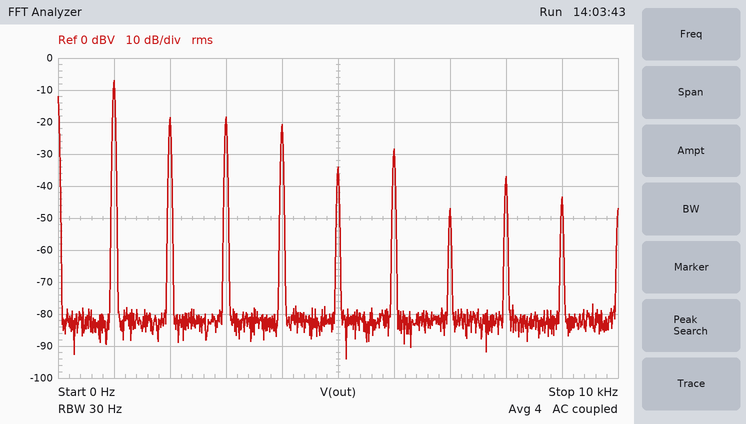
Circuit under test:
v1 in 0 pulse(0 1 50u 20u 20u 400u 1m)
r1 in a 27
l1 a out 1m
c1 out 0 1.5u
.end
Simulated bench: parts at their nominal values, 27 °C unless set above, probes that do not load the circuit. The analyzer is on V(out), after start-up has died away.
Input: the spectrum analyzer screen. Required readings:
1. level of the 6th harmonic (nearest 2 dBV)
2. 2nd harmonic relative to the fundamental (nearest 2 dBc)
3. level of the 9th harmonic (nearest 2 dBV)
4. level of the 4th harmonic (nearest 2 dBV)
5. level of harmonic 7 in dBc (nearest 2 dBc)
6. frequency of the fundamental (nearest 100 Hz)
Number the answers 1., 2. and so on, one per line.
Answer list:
1. -28 dBV
2. -12 dBc
3. -44 dBV
4. -20 dBV
5. -40 dBc
6. 1.0 kHz
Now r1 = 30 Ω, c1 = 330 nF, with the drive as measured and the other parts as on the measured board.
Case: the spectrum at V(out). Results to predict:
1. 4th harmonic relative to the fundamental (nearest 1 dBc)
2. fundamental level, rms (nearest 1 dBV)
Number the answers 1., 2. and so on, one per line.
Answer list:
1. -12 dBc
2. -7 dBV
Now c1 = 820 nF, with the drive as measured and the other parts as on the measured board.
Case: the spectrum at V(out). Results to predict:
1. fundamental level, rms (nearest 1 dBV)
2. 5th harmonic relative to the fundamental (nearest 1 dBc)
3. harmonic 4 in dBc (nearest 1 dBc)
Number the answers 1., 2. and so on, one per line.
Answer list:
1. -7 dBV
2. -21 dBc
3. -11 dBc
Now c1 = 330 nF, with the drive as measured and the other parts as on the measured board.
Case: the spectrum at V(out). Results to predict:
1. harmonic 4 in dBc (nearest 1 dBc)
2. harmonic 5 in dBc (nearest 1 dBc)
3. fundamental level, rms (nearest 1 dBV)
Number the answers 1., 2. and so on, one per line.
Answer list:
1. -12 dBc
2. -21 dBc
3. -7 dBV
